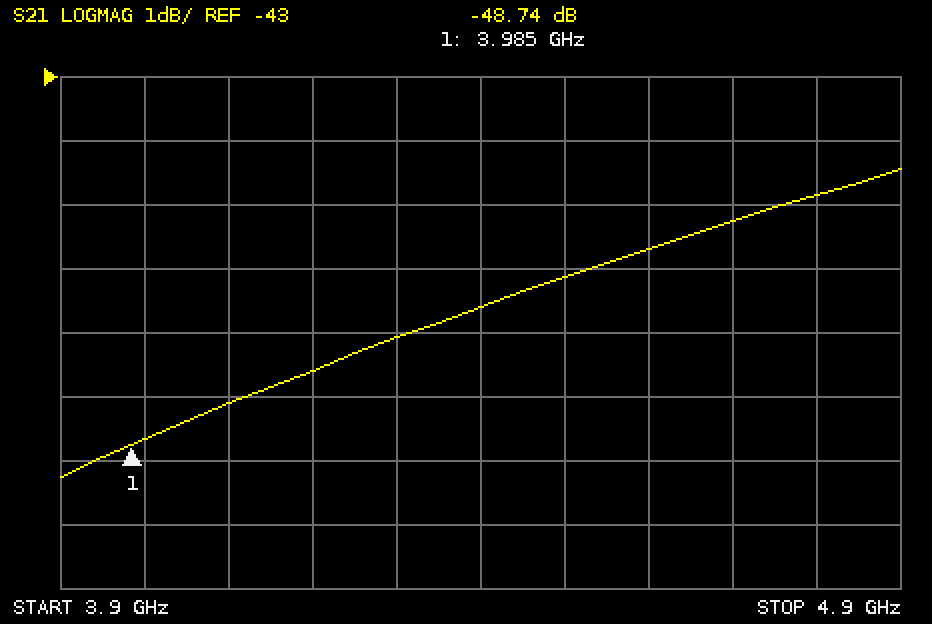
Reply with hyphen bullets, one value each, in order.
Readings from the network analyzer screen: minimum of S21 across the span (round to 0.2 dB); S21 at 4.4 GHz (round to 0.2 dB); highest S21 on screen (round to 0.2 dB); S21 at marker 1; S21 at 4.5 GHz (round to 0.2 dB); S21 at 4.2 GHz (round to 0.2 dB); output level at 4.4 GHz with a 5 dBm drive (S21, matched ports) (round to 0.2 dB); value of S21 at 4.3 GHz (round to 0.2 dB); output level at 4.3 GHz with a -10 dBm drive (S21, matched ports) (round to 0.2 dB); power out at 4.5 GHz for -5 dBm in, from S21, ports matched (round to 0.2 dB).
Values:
- -49.2 dB
- -46.6 dB
- -44.4 dB
- -48.74 dB
- -46.2 dB
- -47.6 dB
- -41.6 dBm
- -47.0 dB
- -57.0 dBm
- -51.2 dBm
